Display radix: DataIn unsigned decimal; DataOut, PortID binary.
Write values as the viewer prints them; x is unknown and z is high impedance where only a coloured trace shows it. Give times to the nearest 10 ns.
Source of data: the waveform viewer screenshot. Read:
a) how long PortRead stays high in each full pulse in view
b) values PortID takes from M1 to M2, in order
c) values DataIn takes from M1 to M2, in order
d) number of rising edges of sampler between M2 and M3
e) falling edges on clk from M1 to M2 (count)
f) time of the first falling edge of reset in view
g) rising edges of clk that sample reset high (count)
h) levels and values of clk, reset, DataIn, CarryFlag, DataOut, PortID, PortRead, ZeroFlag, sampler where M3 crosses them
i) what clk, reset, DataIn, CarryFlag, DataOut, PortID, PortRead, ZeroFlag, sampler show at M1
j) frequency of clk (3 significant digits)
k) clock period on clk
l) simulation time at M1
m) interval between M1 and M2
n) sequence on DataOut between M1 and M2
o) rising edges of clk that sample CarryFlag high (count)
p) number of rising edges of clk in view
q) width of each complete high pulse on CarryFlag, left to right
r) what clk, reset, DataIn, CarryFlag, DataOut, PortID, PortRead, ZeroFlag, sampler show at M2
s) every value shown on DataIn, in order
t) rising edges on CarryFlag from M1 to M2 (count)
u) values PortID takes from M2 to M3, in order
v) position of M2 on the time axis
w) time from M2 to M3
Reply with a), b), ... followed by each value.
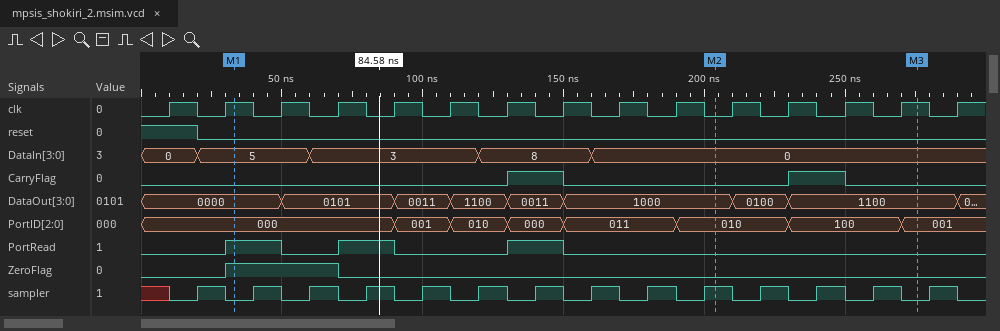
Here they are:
a) 20 ns, 20 ns, 20 ns
b) 000, 001, 010, 000, 011, 010
c) 5, 3, 8, 0
d) 3
e) 9
f) 20 ns
g) 1
h) clk=1, reset=0, DataIn=0, CarryFlag=0, DataOut=1100, PortID=001, PortRead=0, ZeroFlag=0, sampler=0
i) clk=1, reset=0, DataIn=5, CarryFlag=0, DataOut=0000, PortID=000, PortRead=1, ZeroFlag=1, sampler=0
j) 50.0 MHz
k) 20 ns
l) 30 ns
m) 170 ns
n) 0000, 0101, 0011, 1100, 0011, 1000
o) 2
p) 15
q) 20 ns, 20 ns
r) clk=0, reset=0, DataIn=0, CarryFlag=0, DataOut=1000, PortID=010, PortRead=0, ZeroFlag=0, sampler=1
s) 0, 5, 3, 8, 0
t) 1
u) 010, 100, 001
v) 200 ns
w) 70 ns
